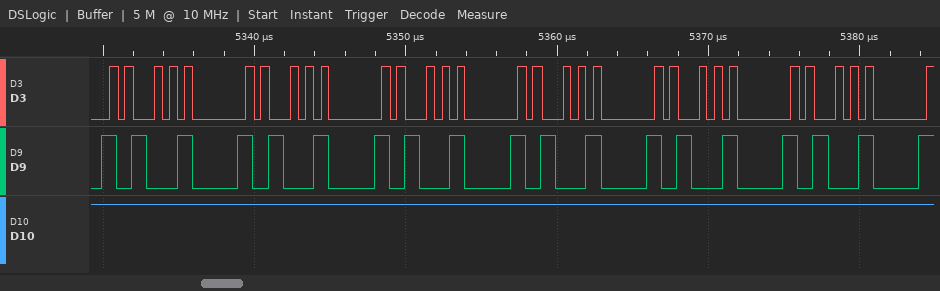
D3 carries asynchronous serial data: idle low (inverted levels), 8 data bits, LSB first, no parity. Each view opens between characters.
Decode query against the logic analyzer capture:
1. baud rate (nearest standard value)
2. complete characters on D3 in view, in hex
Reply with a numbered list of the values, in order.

1. 2000000 baud
2. 5D, 7F, 57, 5D, 7F, 57, 5D, 7F, 57
